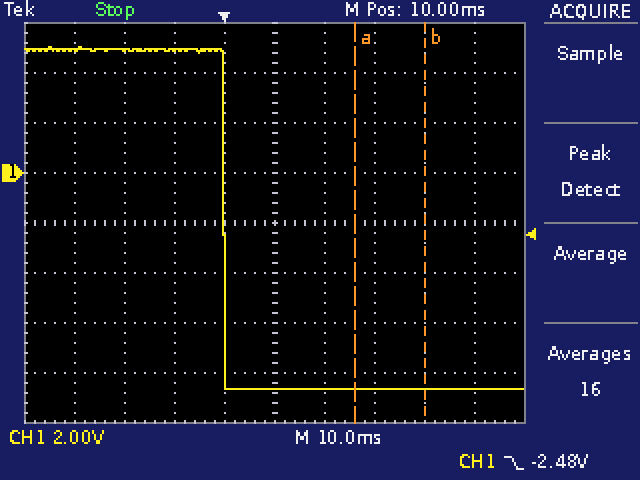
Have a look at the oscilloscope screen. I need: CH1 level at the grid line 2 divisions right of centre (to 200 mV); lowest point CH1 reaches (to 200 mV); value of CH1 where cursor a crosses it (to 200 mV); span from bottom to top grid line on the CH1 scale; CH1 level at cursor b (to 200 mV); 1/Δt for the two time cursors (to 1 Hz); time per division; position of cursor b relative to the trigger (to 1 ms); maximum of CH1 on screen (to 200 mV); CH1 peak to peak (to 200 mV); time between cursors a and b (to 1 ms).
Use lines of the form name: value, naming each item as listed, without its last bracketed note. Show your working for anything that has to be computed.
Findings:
CH1 level at the grid line 2 divisions right of centre: -8.6 V
lowest point CH1 reaches: -8.6 V
value of CH1 where cursor a crosses it: -8.6 V
span from bottom to top grid line on the CH1 scale: 16 V
CH1 level at cursor b: -8.6 V
1/Δt for the two time cursors: 1 / 14 ms ≈ 71 Hz
time per division: 10 ms
position of cursor b relative to the trigger: +40 ms
maximum of CH1 on screen: 5.0 V
CH1 peak to peak: 5.0 V − (-8.6 V) = 13.6 V
time between cursors a and b: 14 ms
